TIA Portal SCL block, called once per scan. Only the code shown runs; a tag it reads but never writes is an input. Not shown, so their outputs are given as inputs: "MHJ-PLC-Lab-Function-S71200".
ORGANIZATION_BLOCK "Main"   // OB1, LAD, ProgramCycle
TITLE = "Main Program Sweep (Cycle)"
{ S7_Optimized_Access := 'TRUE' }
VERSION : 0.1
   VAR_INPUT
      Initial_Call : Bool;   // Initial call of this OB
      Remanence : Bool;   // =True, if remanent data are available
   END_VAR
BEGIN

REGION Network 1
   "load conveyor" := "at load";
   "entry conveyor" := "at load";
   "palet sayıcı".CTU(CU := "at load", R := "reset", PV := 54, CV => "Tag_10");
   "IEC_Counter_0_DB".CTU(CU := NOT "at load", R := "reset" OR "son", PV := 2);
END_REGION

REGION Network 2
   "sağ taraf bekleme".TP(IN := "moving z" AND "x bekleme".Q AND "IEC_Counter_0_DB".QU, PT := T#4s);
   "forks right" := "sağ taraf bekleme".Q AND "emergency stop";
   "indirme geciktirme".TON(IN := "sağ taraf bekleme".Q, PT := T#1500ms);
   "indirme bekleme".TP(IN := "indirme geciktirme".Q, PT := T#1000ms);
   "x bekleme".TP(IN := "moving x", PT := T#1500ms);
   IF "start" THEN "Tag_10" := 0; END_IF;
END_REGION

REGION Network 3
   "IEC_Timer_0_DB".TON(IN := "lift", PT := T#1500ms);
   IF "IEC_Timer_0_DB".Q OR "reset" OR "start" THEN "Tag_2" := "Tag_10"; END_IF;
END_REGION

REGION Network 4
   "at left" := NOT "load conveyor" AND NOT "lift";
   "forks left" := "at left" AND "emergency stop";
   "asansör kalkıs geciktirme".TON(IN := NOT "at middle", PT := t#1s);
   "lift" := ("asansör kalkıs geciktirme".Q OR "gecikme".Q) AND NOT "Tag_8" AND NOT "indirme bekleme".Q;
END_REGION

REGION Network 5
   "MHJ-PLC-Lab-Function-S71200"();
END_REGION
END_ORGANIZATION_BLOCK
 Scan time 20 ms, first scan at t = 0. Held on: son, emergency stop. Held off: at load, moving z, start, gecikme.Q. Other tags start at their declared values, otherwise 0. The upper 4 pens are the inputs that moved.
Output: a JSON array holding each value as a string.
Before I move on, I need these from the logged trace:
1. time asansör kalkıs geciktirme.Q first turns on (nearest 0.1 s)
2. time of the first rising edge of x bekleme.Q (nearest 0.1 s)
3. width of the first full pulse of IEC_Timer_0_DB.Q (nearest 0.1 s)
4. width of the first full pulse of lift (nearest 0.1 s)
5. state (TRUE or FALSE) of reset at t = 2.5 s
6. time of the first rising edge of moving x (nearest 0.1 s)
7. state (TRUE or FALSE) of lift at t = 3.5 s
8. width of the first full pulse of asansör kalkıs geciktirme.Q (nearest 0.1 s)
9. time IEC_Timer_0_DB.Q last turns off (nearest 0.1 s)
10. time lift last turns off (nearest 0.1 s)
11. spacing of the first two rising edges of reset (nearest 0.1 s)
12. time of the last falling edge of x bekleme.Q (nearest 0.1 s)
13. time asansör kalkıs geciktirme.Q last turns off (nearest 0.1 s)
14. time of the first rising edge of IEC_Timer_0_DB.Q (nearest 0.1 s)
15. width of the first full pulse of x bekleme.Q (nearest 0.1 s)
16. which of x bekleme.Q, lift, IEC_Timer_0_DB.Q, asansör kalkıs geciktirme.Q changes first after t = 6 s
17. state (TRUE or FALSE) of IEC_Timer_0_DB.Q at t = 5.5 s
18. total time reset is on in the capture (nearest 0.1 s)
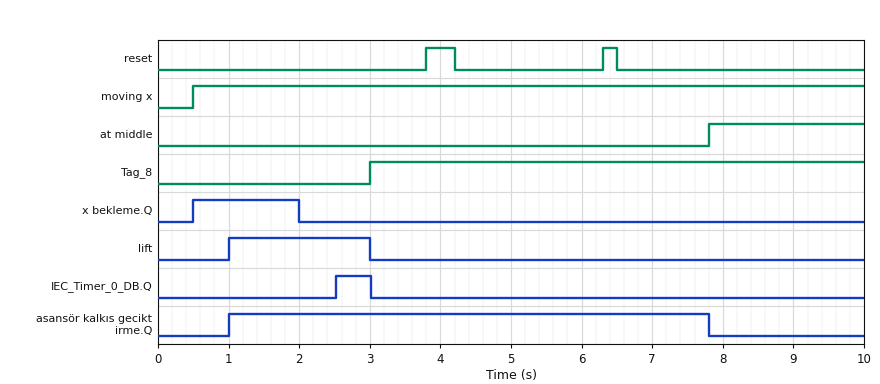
["1.0 s", "0.5 s", "0.5 s", "2.0 s", "FALSE", "0.5 s", "FALSE", "6.8 s", "3.0 s", "3.0 s", "2.5 s", "2.0 s", "7.8 s", "2.5 s", "1.5 s", "asansör kalkıs geciktirme.Q", "FALSE", "0.6 s"]
